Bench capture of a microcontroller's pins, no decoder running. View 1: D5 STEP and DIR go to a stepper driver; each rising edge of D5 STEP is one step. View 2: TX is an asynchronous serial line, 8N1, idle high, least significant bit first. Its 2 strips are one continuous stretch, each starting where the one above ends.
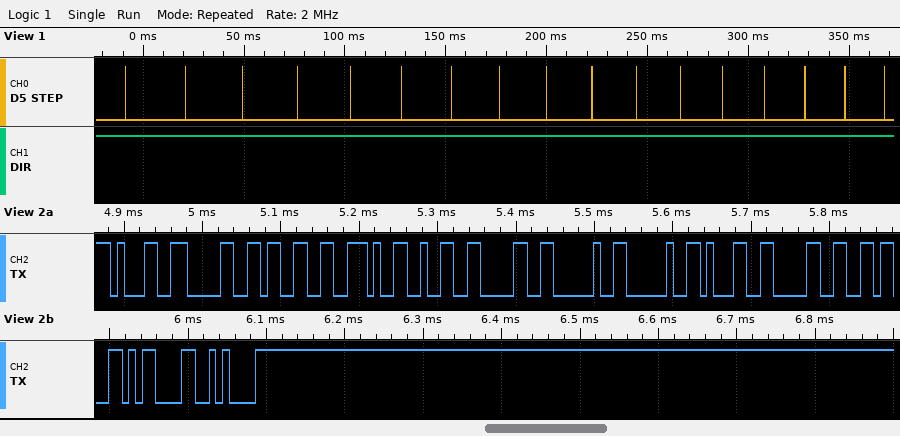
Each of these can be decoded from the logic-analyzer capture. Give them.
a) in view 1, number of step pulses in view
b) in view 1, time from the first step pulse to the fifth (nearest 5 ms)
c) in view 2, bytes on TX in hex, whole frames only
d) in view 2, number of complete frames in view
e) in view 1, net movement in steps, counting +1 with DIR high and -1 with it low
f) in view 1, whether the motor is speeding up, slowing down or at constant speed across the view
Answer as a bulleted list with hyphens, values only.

- 17
- 110 ms
- 31 30 33 2E 32 30 20 20 31 30 36 0D 0A
- 13
- +17
- speeding up
